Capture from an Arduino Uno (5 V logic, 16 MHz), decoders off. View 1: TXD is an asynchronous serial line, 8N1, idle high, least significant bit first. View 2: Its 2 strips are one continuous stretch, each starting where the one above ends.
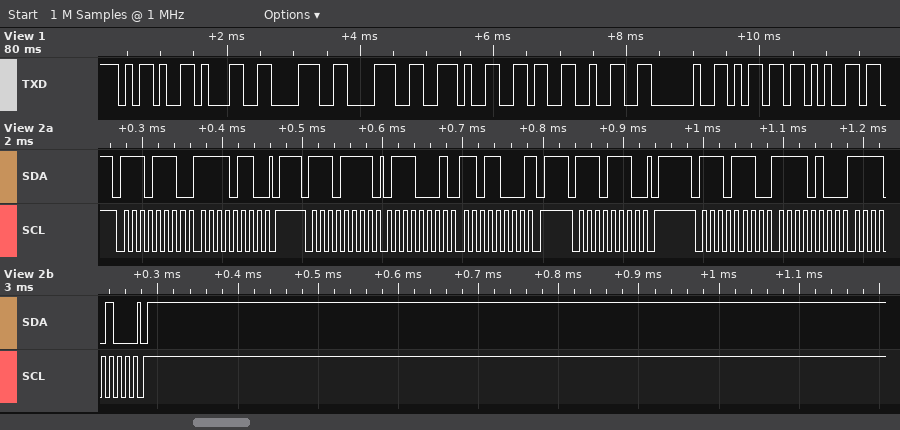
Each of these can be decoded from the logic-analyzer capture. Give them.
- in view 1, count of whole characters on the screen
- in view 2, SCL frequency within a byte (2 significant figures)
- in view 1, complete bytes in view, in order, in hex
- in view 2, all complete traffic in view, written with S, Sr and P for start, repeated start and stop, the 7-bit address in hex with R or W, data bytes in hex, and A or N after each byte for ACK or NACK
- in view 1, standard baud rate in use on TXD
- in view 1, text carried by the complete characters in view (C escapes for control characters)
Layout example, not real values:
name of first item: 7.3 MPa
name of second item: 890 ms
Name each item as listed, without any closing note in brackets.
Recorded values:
in view 1, count of whole characters on the screen: 10
in view 2, SCL frequency within a byte: 100 kHz
in view 1, complete bytes in view, in order, in hex: 0x2D 0x31 0x38 0x38 0x2E 0x36 0x32 0x20 0x6D 0x65
in view 2, all complete traffic in view, written with S, Sr and P for start, repeated start and stop, the 7-bit address in hex with R or W, data bytes in hex, and A or N after each byte for ACK or NACK: S 77W A F6 A P S 77R A 71 A D8 N P S 77W A P S 77W A F4 A F4 A P
in view 1, standard baud rate in use on TXD: 9600 baud
in view 1, text carried by the complete characters in view: "-188.62 me"
